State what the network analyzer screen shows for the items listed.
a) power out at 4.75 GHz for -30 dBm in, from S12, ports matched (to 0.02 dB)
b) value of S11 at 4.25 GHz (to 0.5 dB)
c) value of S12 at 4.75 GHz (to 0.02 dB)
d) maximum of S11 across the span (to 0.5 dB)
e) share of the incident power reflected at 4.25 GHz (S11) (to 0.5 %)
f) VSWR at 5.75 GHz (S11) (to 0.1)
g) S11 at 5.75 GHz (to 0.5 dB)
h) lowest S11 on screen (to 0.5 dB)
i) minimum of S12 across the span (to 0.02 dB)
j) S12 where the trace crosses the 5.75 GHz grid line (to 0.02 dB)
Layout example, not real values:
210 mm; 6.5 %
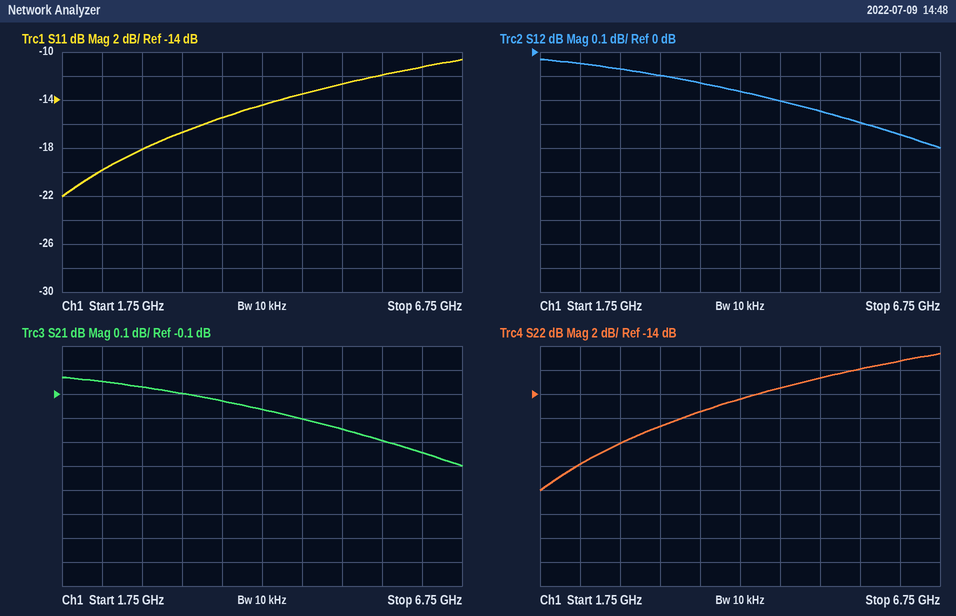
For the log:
-30.20 dBm; -14.5 dB; -0.20 dB; -10.5 dB; 3.5 %; 1.7; -12.0 dB; -22.0 dB; -0.40 dB; -0.30 dB
